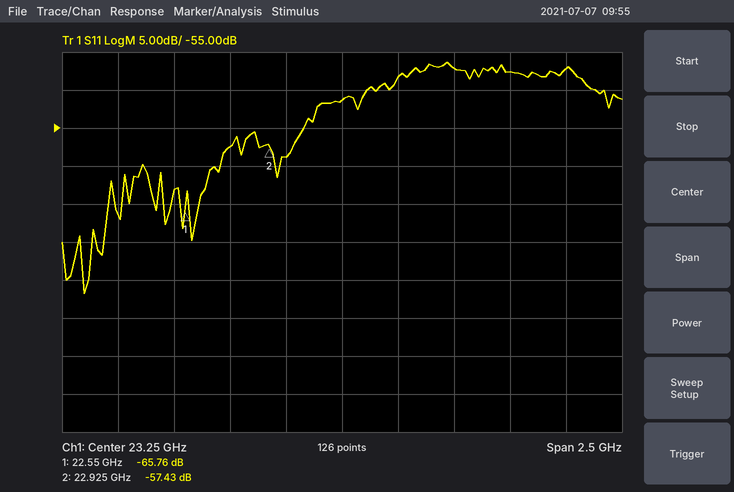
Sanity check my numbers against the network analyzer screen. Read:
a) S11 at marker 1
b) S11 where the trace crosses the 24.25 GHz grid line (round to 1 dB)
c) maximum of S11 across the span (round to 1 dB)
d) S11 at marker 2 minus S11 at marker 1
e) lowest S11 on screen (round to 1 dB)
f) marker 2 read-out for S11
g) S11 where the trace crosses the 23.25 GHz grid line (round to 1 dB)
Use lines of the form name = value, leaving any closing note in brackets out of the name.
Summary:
S11 at marker 1 = -65.76 dB
S11 where the trace crosses the 24.25 GHz grid line = -47 dB
maximum of S11 across the span = -46 dB
S11 at marker 2 minus S11 at marker 1 = 8.33 dB
lowest S11 on screen = -77 dB
marker 2 read-out for S11 = -57.43 dB
S11 where the trace crosses the 23.25 GHz grid line = -51 dB
